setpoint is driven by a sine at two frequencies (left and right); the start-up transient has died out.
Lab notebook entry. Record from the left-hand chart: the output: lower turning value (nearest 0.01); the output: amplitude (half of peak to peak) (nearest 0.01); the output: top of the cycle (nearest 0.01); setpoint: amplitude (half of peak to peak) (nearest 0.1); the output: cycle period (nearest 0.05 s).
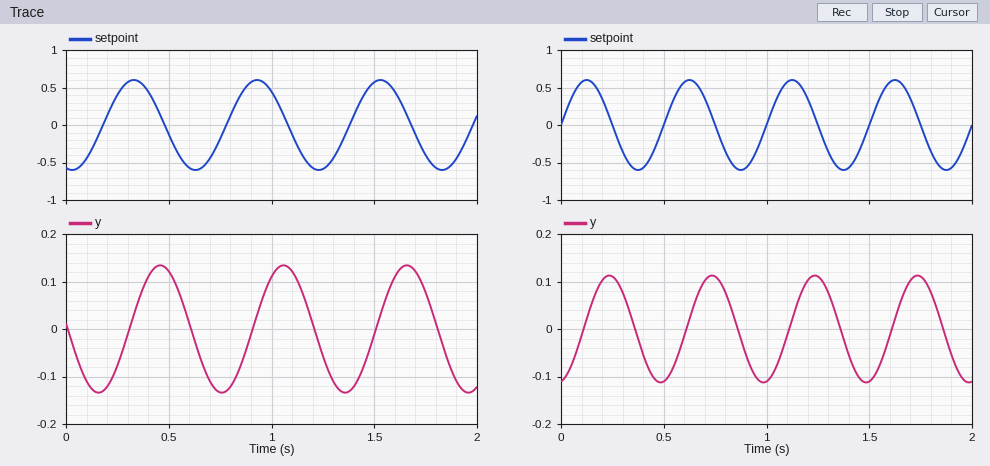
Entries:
-0.13
0.13
0.13
0.6
0.60 s
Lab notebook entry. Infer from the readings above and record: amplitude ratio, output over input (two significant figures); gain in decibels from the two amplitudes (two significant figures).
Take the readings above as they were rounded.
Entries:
0.22
-13 dB
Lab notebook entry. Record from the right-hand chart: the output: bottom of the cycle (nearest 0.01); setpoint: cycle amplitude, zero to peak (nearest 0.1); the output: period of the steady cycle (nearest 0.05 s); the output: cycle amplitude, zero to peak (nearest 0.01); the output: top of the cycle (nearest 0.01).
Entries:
-0.11
0.6
0.50 s
0.11
0.11
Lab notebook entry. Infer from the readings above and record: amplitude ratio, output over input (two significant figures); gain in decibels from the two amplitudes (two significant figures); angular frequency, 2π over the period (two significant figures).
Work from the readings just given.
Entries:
0.18
-15 dB
13 rad/s
